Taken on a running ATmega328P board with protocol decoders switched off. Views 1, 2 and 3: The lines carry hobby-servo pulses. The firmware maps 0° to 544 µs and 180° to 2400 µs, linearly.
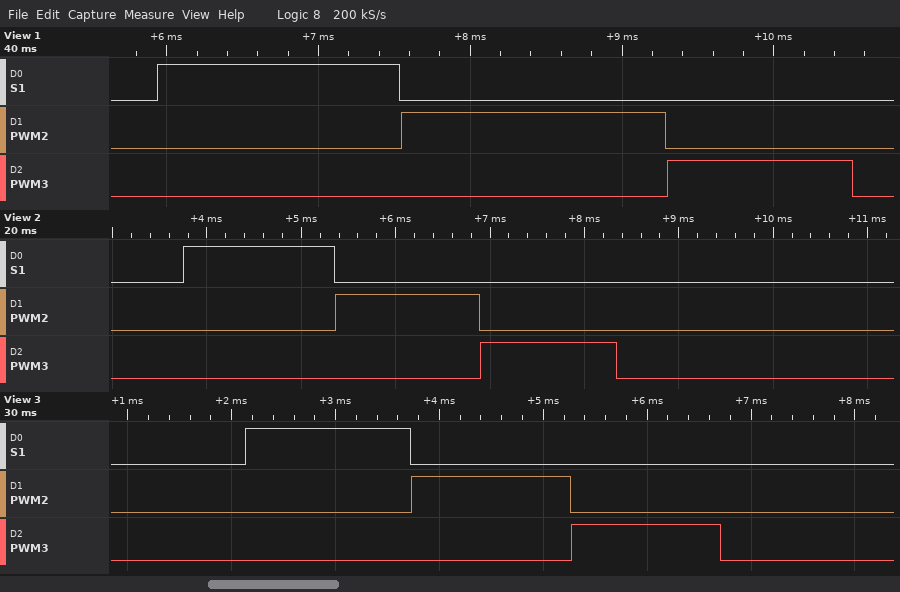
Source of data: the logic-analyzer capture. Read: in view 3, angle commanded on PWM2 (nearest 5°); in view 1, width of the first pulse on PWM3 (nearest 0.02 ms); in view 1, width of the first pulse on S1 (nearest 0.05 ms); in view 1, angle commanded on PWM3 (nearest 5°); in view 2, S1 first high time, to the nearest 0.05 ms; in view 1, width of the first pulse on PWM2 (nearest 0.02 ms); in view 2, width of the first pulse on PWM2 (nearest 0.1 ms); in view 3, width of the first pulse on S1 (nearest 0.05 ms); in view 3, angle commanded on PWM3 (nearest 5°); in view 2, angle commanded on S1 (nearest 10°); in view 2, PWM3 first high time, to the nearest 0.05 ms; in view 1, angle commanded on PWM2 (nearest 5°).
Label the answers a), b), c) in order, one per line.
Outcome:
a) 95°
b) 1.22 ms
c) 1.60 ms
d) 65°
e) 1.60 ms
f) 1.74 ms
g) 1.5 ms
h) 1.60 ms
i) 85°
j) 100°
k) 1.45 ms
l) 115°
